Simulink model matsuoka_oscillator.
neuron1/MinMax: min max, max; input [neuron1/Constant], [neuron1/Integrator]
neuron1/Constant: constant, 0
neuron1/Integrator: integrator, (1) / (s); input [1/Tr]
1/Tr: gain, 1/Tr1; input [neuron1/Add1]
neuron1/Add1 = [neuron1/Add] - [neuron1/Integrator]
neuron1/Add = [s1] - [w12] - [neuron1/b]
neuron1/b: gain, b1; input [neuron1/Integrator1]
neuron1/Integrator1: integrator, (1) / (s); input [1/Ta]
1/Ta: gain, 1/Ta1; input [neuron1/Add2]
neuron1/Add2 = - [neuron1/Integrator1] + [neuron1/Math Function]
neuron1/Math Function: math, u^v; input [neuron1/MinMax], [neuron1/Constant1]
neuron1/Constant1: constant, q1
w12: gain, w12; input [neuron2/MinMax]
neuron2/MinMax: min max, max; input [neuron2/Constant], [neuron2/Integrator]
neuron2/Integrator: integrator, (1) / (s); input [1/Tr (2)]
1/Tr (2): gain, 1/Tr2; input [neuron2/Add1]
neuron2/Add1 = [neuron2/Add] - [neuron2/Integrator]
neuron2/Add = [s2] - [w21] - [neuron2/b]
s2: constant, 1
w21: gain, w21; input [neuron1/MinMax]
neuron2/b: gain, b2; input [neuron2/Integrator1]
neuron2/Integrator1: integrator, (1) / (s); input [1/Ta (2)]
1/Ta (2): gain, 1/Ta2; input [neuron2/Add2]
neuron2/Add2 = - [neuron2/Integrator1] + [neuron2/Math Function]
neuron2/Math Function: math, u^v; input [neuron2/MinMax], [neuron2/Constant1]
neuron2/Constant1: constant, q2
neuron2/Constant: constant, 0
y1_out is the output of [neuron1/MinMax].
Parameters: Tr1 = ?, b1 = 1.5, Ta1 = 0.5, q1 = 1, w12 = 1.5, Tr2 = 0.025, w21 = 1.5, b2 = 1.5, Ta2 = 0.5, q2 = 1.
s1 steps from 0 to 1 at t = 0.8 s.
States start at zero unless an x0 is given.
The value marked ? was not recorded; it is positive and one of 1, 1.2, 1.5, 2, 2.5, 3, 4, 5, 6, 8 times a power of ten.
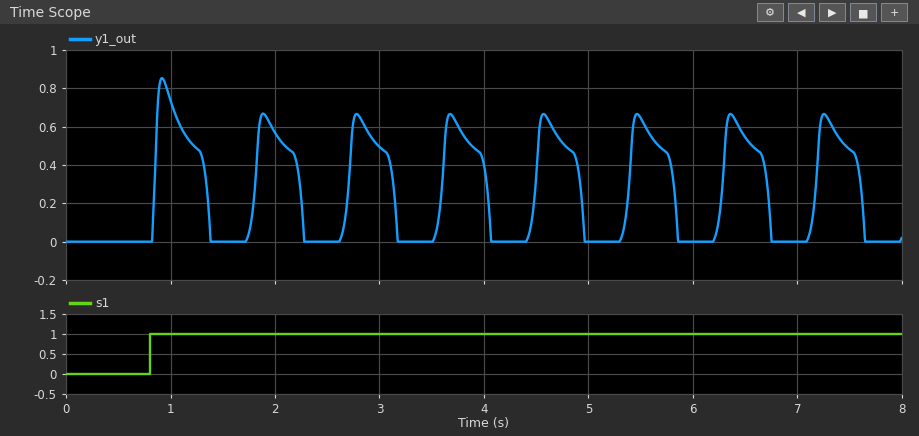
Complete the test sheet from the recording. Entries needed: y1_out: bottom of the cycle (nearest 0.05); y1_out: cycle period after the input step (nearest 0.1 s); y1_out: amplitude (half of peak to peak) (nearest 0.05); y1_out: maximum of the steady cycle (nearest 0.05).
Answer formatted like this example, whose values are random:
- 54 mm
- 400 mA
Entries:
- 0.00
- 0.9 s
- 0.35
- 0.65
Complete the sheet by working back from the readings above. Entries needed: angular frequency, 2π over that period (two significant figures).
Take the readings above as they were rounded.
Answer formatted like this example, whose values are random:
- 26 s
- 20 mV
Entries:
- 7.0 rad/s
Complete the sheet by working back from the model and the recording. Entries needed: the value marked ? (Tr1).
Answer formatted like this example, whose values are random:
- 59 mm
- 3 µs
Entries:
- 0.025
